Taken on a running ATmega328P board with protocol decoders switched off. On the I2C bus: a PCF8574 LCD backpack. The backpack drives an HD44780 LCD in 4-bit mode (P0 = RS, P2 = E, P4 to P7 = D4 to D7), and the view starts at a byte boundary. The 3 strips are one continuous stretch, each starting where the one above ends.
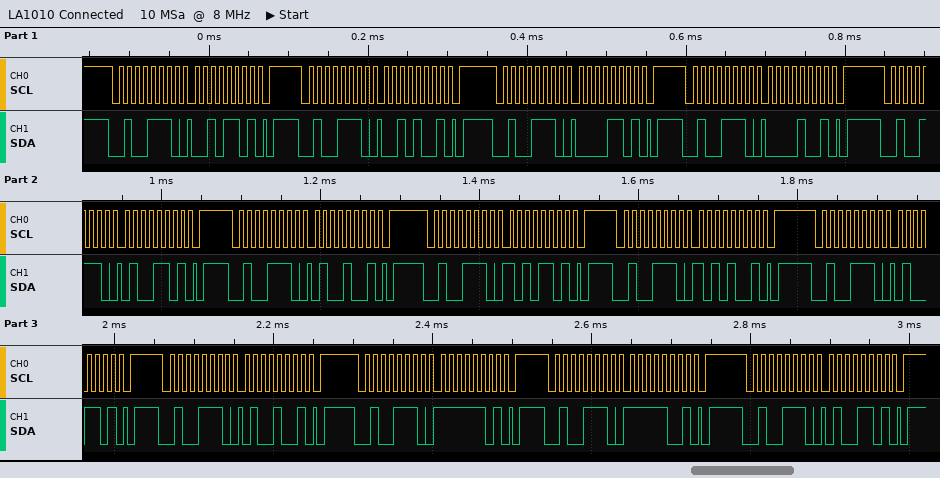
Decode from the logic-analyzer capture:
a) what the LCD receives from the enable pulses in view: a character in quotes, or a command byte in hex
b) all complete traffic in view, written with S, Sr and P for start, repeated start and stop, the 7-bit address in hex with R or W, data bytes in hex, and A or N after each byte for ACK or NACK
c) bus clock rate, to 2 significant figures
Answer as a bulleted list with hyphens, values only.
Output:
- ' ' 'J' 'O'
- S 27W A 2D A P S 27W A 29 A P S 27W A 0D A P S 27W A 09 A P S 27W A 4D A P S 27W A 49 A P S 27W A AD A P S 27W A A9 A P S 27W A 4D A P S 27W A 49 A P S 27W A FD A P S 27W A F9 A P S 27W A 4D A P
- 100 kHz
